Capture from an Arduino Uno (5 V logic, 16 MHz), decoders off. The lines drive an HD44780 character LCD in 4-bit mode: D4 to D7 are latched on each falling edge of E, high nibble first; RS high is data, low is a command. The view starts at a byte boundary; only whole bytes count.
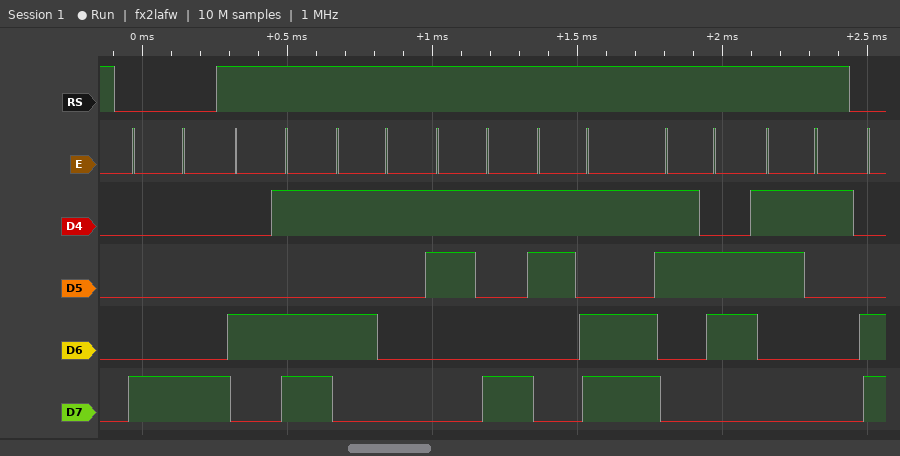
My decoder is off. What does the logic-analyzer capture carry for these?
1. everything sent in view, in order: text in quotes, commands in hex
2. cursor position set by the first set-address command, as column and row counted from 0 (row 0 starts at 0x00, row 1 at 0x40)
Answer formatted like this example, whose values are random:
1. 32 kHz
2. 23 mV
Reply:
1. 0x88 "MQ9=61"
2. column 8, row 0
